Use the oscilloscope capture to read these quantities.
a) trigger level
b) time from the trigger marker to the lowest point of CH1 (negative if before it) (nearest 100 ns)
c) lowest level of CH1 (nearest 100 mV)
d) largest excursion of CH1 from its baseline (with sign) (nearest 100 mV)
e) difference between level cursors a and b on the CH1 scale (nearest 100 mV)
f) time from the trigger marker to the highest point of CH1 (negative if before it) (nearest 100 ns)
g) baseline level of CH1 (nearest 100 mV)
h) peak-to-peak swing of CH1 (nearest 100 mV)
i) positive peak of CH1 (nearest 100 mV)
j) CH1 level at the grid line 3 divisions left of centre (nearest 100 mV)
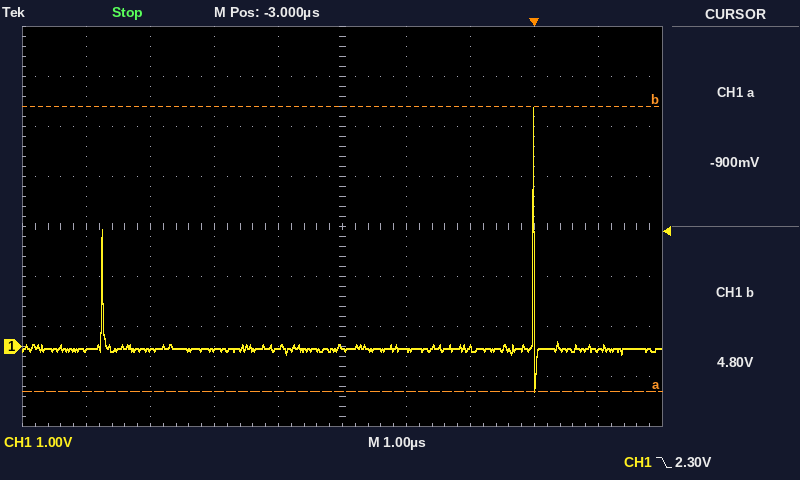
2.30 V
0.0 µs
-900 mV
+4.8 V
5.7 V
0.0 µs
0.0 V
5.7 V
4.8 V
-100 mV
